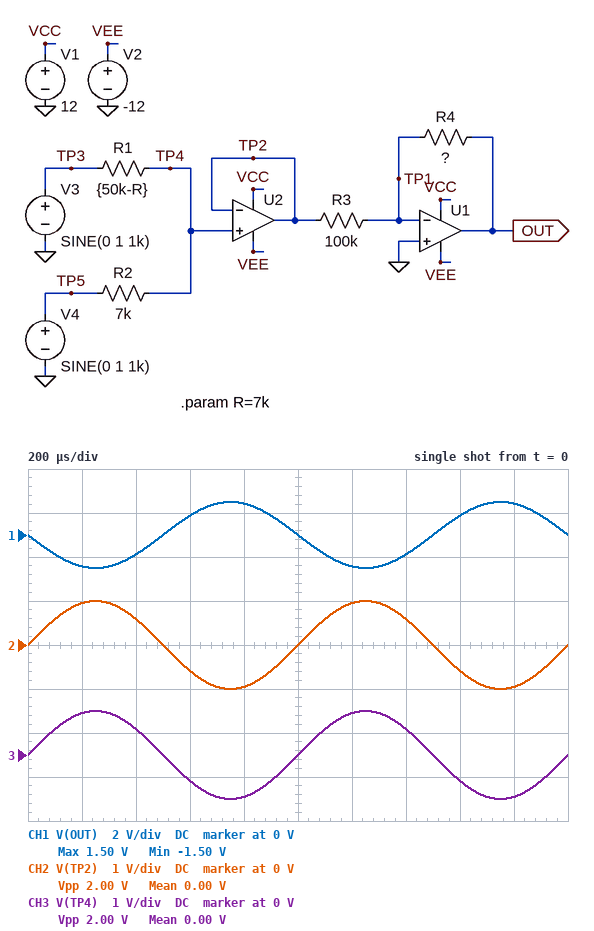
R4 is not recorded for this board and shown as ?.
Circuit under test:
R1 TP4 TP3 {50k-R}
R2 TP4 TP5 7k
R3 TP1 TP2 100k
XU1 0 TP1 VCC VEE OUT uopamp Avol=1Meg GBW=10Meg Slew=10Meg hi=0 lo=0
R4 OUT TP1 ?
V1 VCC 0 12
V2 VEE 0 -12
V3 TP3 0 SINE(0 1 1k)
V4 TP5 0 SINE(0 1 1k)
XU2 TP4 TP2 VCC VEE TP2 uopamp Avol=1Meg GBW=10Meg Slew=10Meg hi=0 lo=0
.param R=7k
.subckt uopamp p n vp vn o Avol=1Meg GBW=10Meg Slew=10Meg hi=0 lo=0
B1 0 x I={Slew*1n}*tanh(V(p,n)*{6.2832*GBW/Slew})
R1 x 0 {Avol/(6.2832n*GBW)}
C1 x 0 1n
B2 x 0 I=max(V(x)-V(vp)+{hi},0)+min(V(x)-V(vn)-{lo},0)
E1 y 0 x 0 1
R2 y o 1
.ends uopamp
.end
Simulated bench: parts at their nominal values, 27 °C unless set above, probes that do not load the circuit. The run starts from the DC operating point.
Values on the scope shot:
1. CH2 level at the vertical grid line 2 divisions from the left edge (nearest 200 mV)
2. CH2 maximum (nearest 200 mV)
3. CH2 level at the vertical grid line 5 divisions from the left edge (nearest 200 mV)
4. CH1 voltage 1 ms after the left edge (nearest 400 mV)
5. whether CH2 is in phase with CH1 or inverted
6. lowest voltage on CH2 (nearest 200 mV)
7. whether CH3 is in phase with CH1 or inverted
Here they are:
600 mV
1.0 V
0 V
0 V
inverted
-1.0 V
inverted
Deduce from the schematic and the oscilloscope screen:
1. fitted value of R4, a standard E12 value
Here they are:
150 kΩ
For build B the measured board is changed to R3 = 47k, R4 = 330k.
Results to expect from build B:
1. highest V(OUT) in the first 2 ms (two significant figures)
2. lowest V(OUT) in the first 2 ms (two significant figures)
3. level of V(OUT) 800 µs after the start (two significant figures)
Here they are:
7.0 V
-7.0 V
6.7 V
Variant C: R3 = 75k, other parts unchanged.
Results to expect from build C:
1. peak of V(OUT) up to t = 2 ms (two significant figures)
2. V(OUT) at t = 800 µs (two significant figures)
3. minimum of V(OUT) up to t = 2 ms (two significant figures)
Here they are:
2.0 V
1.9 V
-2.0 V
